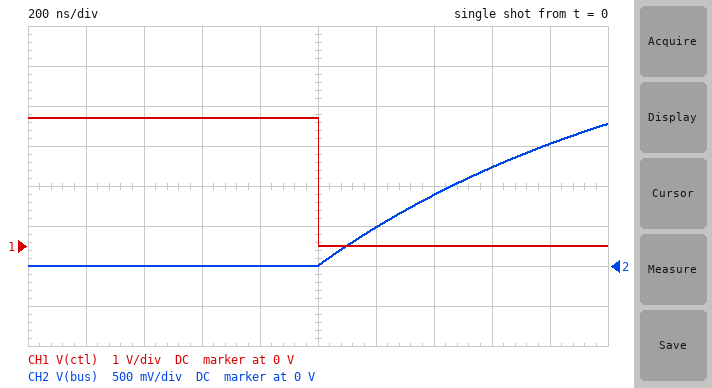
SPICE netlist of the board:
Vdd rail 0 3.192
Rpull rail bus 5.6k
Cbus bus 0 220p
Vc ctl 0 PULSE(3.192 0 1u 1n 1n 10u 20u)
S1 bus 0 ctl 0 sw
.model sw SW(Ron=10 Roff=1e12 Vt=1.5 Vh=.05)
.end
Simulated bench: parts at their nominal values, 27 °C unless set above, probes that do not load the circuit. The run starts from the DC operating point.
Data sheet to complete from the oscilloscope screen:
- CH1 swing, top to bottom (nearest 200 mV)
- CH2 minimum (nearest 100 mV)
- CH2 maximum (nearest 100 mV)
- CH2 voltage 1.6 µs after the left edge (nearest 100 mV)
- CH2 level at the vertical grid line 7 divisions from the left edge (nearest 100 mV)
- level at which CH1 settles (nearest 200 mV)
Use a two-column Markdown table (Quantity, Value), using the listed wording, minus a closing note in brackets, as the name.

| Quantity | Value |
|---|---|
| CH1 swing, top to bottom | 3.2 V |
| CH2 minimum | 0 V |
| CH2 maximum | 1.8 V |
| CH2 voltage 1.6 µs after the left edge | 1.2 V |
| CH2 level at the vertical grid line 7 divisions from the left edge | 900 mV |
| level at which CH1 settles | 0 V |
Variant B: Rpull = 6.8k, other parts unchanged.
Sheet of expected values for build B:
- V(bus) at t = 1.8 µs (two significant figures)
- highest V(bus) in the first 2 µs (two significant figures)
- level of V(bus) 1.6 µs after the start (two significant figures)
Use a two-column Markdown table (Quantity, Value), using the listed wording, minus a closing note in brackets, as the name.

| Quantity | Value |
|---|---|
| V(bus) at t = 1.8 µs | 1.3 V |
| highest V(bus) in the first 2 µs | 1.6 V |
| level of V(bus) 1.6 µs after the start | 1.1 V |
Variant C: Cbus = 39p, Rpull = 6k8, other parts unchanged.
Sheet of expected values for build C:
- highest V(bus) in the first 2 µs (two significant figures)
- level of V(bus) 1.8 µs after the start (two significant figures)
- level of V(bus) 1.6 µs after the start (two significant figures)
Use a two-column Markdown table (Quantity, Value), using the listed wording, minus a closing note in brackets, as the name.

| Quantity | Value |
|---|---|
| highest V(bus) in the first 2 µs | 3.1 V |
| level of V(bus) 1.8 µs after the start | 3.0 V |
| level of V(bus) 1.6 µs after the start | 2.9 V |
